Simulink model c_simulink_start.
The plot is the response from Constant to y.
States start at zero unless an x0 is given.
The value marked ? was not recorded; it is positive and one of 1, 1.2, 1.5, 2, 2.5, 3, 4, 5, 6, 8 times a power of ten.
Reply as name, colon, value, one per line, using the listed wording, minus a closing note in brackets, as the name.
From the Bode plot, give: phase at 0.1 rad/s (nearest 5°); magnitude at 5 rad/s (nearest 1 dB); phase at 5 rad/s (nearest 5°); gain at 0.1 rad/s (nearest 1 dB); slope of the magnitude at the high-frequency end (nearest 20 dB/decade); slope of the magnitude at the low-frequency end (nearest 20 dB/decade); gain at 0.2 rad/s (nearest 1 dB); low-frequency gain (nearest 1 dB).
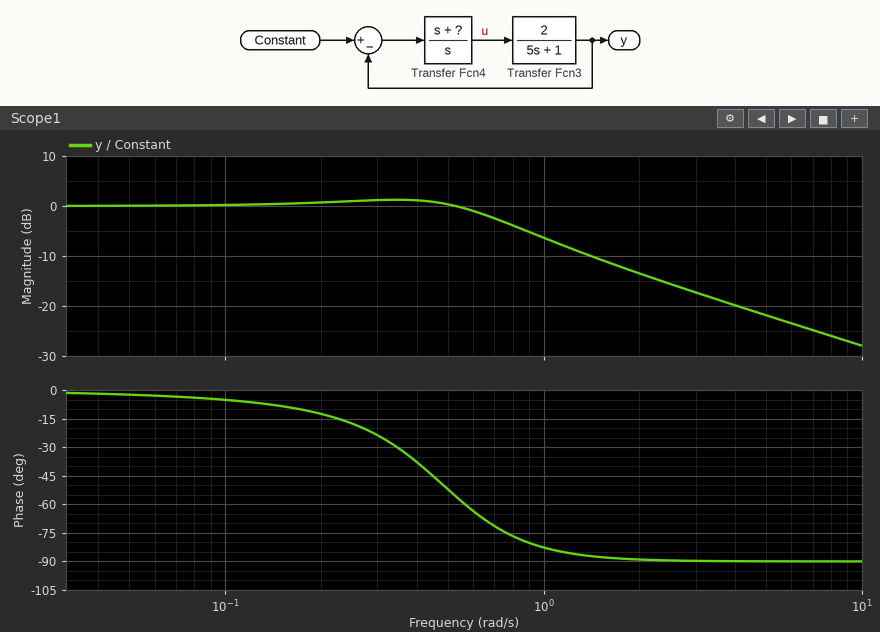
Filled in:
phase at 0.1 rad/s: -5°
magnitude at 5 rad/s: -22 dB
phase at 5 rad/s: -90°
gain at 0.1 rad/s: 0 dB
slope of the magnitude at the high-frequency end: -20 dB/decade
slope of the magnitude at the low-frequency end: 0 dB/decade
gain at 0.2 rad/s: 1 dB
low-frequency gain: 0 dB
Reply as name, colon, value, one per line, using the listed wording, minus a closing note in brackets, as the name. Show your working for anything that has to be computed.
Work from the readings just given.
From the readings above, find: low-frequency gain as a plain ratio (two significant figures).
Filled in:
low-frequency gain as a plain ratio: 10^(0 / 20) = 1.0
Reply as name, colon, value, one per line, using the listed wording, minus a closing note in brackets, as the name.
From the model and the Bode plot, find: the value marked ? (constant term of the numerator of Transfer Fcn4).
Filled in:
the value marked ?: 0.6
